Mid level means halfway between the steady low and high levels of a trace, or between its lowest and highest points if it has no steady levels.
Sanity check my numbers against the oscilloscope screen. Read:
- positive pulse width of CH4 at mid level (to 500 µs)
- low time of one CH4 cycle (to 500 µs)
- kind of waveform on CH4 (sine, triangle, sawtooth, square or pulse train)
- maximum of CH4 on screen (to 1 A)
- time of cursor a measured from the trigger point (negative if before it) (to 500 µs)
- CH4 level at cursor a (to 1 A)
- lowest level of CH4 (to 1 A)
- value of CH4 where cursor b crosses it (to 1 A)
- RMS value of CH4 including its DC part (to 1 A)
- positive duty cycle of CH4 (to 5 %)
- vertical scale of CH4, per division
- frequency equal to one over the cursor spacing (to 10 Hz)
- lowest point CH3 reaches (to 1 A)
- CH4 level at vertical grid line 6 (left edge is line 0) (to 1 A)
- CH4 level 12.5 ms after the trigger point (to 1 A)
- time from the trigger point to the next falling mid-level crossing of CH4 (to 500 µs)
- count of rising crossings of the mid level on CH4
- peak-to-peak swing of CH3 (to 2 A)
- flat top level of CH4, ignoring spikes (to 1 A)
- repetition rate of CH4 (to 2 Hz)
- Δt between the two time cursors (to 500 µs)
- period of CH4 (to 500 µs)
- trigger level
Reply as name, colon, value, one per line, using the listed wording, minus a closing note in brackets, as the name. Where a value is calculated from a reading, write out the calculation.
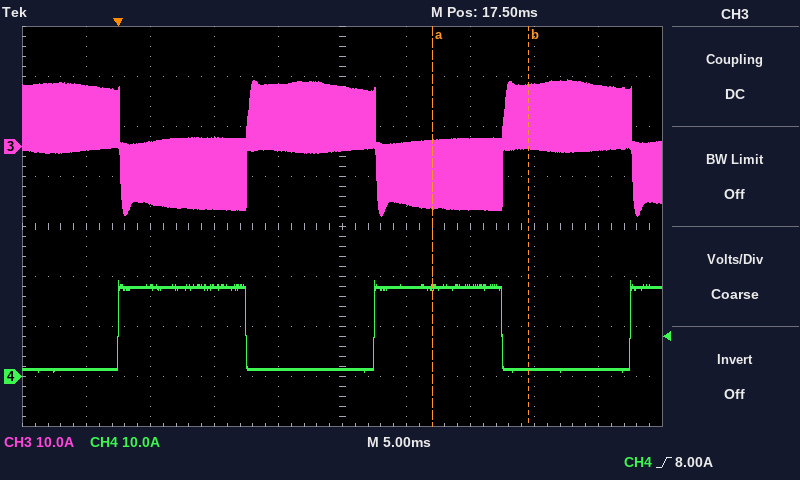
positive pulse width of CH4 at mid level: 10.0 ms
low time of one CH4 cycle: 10.0 ms
kind of waveform on CH4: square
maximum of CH4 on screen: 19 A
time of cursor a measured from the trigger point (negative if before it): +24.5 ms
CH4 level at cursor a: 18 A
lowest level of CH4: 1 A
value of CH4 where cursor b crosses it: 1 A
RMS value of CH4 including its DC part: √(0.5 × (18 A)² + 0.5 × (1 A)²) ≈ 13 A
positive duty cycle of CH4: 10.0 ms / 20.0 ms ≈ 50 %
vertical scale of CH4, per division: 10 A
frequency equal to one over the cursor spacing: 1 / 7.5 ms ≈ 130 Hz
lowest point CH3 reaches: -14 A
CH4 level at vertical grid line 6 (left edge is line 0): 18 A
CH4 level 12.5 ms after the trigger point: 1 A
time from the trigger point to the next falling mid-level crossing of CH4: 10.0 ms
count of rising crossings of the mid level on CH4: 3
peak-to-peak swing of CH3: 28 A
flat top level of CH4, ignoring spikes: 18 A
repetition rate of CH4: 1 / 20.0 ms ≈ 50 Hz
Δt between the two time cursors: 7.5 ms
period of CH4: 20.0 ms
trigger level: 8.00 A
